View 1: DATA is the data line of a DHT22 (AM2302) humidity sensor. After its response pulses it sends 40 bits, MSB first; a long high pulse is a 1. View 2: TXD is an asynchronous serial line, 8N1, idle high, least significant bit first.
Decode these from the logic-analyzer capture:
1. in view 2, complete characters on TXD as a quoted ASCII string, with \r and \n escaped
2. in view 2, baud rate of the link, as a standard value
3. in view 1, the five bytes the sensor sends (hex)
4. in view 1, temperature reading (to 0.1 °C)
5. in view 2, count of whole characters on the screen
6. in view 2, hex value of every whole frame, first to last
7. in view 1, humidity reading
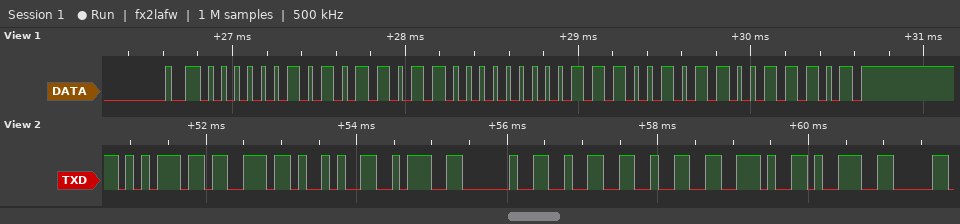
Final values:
"us): 22.9"
9600 baud
02 B6 00 E5 9D
22.9 °C
9
0x75 0x73 0x29 0x3A 0x20 0x32 0x32 0x2E 0x39
69.4 %
